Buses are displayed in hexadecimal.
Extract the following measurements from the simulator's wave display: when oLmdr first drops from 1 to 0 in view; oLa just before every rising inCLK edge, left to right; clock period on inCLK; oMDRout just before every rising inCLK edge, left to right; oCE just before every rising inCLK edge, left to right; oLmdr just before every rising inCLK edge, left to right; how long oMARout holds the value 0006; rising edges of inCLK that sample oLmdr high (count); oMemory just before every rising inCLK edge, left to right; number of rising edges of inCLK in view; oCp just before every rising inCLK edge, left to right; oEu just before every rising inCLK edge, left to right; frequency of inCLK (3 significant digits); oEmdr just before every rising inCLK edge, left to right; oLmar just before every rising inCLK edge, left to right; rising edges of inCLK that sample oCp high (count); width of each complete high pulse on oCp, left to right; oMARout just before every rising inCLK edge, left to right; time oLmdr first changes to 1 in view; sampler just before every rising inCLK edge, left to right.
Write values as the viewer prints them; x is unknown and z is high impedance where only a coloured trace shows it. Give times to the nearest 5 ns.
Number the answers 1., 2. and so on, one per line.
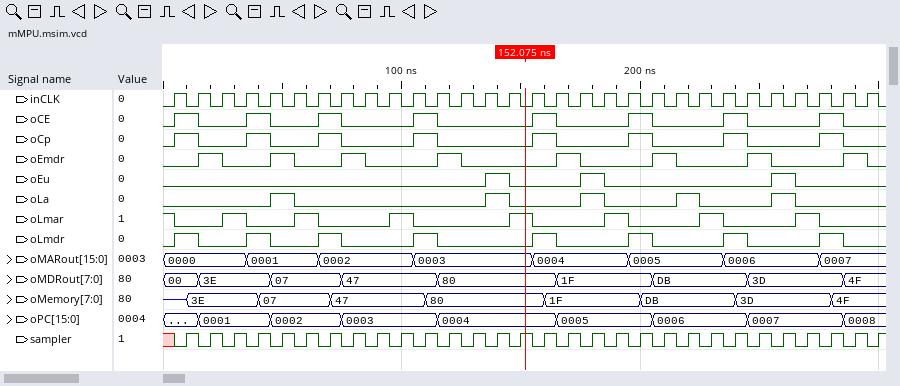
1. 15 ns
2. 0 0 0 0 0 1 0 0 0 0 0 0 0 0 1 0 0 0 1 0 0 0 1 0 0 0 1 0 0 0
3. 10 ns
4. 00, 00, 3E, 3E, 3E, 07, 07, 07, 47, 47, 47, 47, 80, 80, 80, 80, 80, 1F, 1F, 1F, 1F, DB, DB, DB, DB, 3D, 3D, 3D, 3D, 4F
5. 0 1 0 0 1 0 0 1 0 0 0 1 0 0 0 0 1 0 0 0 1 0 0 0 1 0 0 0 1 0
6. 0 1 0 0 1 0 0 1 0 0 0 1 0 0 0 0 1 0 0 0 1 0 0 0 1 0 0 0 1 0
7. 40 ns
8. 8
9. z, 3E, 3E, 3E, 07, 07, 07, 47, 47, 47, 47, 80, 80, 80, 80, 80, 1F, 1F, 1F, 1F, DB, DB, DB, DB, 3D, 3D, 3D, 3D, 4F, 4F
10. 30
11. 0 1 0 0 1 0 0 1 0 0 0 1 0 0 0 0 1 0 0 0 1 0 0 0 1 0 0 0 1 0
12. 0 0 0 0 0 0 0 0 0 0 0 0 0 0 1 0 0 0 1 0 0 0 0 0 0 0 1 0 0 0
13. 100 MHz
14. 0 0 1 0 0 1 0 0 1 0 0 0 1 0 0 0 0 1 0 0 0 1 0 0 0 1 0 0 0 1
15. 1 0 0 1 0 0 1 0 0 0 1 0 0 0 0 1 0 0 0 1 0 0 0 1 0 0 0 1 0 0
16. 8
17. 10 ns, 10 ns, 10 ns, 10 ns, 10 ns, 10 ns, 10 ns, 10 ns
18. 0000, 0000, 0000, 0000, 0001, 0001, 0001, 0002, 0002, 0002, 0002, 0003, 0003, 0003, 0003, 0003, 0004, 0004, 0004, 0004, 0005, 0005, 0005, 0005, 0006, 0006, 0006, 0006, 0007, 0007
19. 5 ns
20. x 1 1 1 1 1 1 1 1 1 1 1 1 1 1 1 1 1 1 1 1 1 1 1 1 1 1 1 1 1
